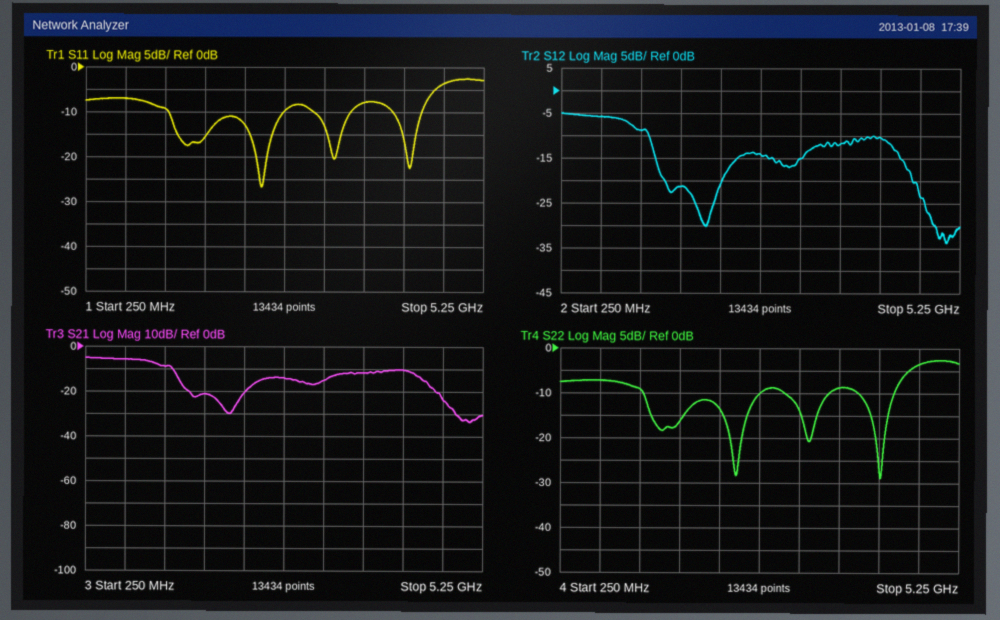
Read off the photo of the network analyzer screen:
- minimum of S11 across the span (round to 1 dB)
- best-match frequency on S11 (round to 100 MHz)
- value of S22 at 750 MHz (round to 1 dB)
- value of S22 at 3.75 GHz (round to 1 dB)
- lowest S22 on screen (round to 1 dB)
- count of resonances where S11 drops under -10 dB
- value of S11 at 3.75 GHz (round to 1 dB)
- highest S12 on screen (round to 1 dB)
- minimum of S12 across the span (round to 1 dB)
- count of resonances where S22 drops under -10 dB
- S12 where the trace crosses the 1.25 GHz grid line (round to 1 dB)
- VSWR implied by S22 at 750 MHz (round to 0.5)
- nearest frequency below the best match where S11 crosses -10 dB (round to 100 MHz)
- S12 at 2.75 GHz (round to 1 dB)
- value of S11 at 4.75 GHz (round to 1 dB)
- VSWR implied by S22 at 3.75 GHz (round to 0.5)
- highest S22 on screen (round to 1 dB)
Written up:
-27 dB
2.5 GHz
-7 dB
-9 dB
-29 dB
4
-8 dB
-5 dB
-34 dB
4
-9 dB
2.5
1.3 GHz
-14 dB
-4 dB
2.0
-3 dB
